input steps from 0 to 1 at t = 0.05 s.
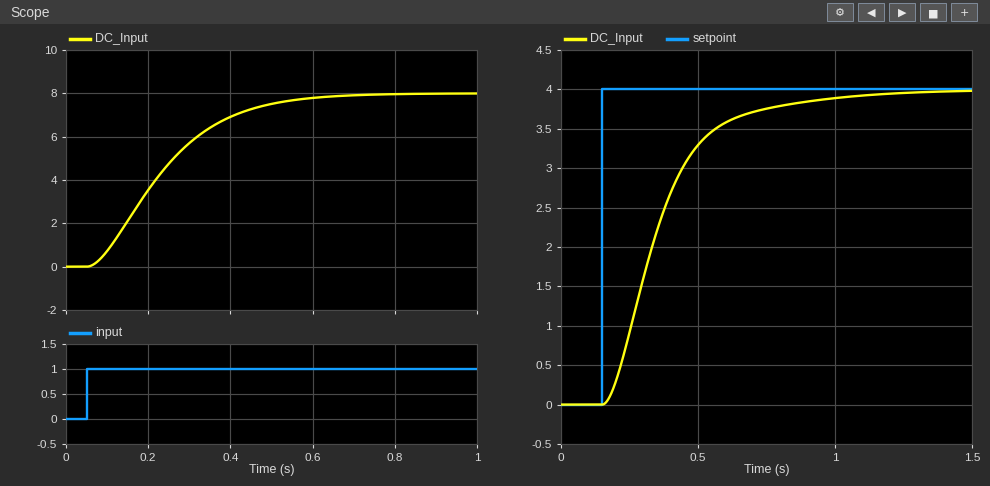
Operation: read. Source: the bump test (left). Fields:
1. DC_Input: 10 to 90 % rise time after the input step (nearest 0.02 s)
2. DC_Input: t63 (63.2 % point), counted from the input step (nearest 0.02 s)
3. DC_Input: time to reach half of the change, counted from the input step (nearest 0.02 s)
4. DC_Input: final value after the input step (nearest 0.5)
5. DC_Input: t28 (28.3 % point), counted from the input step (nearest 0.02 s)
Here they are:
0.34 s
0.22 s
0.16 s
8.0
0.10 s
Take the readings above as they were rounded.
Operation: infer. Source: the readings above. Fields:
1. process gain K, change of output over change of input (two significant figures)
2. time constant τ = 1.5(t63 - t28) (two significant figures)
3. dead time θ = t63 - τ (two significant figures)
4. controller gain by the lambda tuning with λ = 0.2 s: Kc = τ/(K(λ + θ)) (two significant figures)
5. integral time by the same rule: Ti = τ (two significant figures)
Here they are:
8.0
0.18 s
0.040 s
0.094
0.18 s
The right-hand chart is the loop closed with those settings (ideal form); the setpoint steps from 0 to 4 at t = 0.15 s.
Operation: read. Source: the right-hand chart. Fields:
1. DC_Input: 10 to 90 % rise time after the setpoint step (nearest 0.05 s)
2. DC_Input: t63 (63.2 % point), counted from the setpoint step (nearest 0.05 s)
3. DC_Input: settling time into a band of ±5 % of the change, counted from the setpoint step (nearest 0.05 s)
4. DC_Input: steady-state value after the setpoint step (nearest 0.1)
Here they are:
0.40 s
0.25 s
0.65 s
4.0
